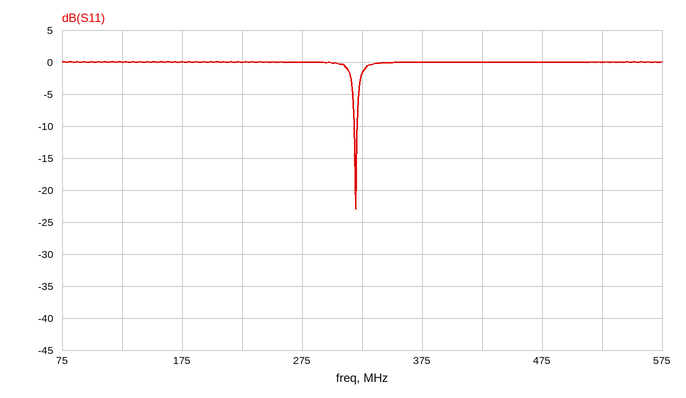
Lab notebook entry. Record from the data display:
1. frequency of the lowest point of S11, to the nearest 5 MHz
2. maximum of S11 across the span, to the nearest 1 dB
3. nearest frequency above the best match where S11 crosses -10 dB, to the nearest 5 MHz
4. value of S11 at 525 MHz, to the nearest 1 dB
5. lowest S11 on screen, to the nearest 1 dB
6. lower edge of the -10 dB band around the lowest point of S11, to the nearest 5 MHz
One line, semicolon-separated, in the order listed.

320 MHz; 0 dB; 320 MHz; 0 dB; -23 dB; 320 MHz
